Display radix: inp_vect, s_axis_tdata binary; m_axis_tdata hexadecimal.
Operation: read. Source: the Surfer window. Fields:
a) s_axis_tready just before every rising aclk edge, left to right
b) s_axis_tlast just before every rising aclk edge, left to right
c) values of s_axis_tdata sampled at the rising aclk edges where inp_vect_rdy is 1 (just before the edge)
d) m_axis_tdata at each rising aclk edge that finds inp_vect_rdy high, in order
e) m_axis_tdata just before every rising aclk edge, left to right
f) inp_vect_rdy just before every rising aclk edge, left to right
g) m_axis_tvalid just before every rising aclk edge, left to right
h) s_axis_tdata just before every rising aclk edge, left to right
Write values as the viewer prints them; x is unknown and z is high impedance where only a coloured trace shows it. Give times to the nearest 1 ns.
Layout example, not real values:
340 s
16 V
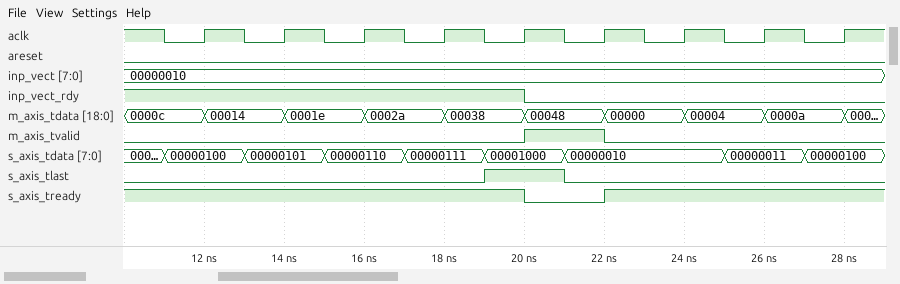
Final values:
1 1 1 1 1 0 1 1 1
0 0 0 0 1 0 0 0 0
00000100, 00000101, 00000110, 00000111, 00001000
0000c, 00014, 0001e, 0002a, 00038
0000c, 00014, 0001e, 0002a, 00038, 00048, 00000, 00004, 0000a
1 1 1 1 1 0 0 0 0
0 0 0 0 0 1 0 0 0
00000100, 00000101, 00000110, 00000111, 00001000, 00000010, 00000010, 00000011, 00000100
